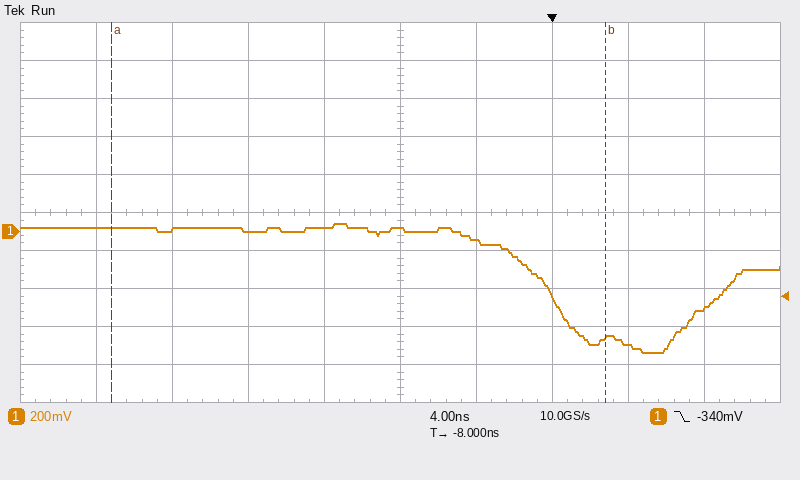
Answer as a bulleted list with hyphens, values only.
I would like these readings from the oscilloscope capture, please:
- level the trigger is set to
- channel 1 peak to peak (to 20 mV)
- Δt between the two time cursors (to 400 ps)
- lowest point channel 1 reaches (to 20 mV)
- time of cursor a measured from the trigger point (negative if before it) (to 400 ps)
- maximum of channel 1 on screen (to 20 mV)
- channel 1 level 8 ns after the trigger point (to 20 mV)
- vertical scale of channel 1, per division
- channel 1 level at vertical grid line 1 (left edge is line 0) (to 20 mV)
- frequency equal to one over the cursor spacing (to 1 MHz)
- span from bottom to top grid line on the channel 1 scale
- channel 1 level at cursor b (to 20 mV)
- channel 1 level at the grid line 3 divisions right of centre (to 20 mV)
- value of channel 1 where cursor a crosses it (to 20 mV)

- -340 mV
- 680 mV
- 26.0 ns
- -640 mV
- -23.2 ns
- 40 mV
- -400 mV
- 200 mV
- 20 mV
- 38 MHz
- 2 V
- -560 mV
- -600 mV
- 20 mV
